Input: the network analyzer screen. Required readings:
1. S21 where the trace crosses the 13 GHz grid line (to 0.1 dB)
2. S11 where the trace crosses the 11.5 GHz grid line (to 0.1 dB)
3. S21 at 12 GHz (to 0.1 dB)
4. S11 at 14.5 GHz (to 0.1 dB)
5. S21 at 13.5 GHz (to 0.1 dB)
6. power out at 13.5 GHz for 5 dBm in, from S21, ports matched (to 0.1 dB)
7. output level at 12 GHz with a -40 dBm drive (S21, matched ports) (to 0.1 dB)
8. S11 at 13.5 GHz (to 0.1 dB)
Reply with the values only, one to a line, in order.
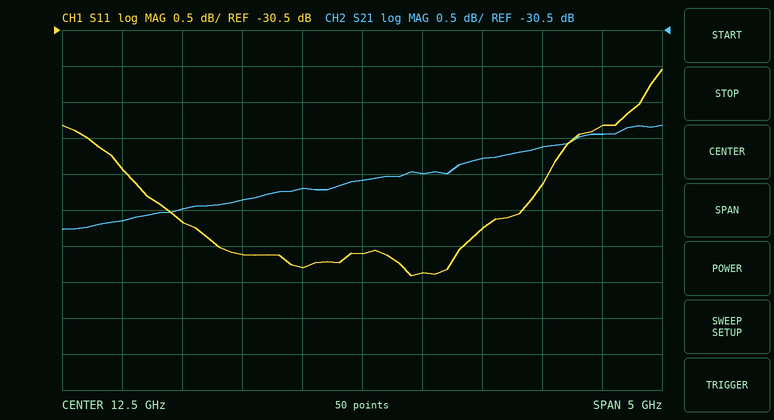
-32.5 dB
-33.6 dB
-32.7 dB
-31.8 dB
-32.3 dB
-27.3 dBm
-72.7 dBm
-33.3 dB
